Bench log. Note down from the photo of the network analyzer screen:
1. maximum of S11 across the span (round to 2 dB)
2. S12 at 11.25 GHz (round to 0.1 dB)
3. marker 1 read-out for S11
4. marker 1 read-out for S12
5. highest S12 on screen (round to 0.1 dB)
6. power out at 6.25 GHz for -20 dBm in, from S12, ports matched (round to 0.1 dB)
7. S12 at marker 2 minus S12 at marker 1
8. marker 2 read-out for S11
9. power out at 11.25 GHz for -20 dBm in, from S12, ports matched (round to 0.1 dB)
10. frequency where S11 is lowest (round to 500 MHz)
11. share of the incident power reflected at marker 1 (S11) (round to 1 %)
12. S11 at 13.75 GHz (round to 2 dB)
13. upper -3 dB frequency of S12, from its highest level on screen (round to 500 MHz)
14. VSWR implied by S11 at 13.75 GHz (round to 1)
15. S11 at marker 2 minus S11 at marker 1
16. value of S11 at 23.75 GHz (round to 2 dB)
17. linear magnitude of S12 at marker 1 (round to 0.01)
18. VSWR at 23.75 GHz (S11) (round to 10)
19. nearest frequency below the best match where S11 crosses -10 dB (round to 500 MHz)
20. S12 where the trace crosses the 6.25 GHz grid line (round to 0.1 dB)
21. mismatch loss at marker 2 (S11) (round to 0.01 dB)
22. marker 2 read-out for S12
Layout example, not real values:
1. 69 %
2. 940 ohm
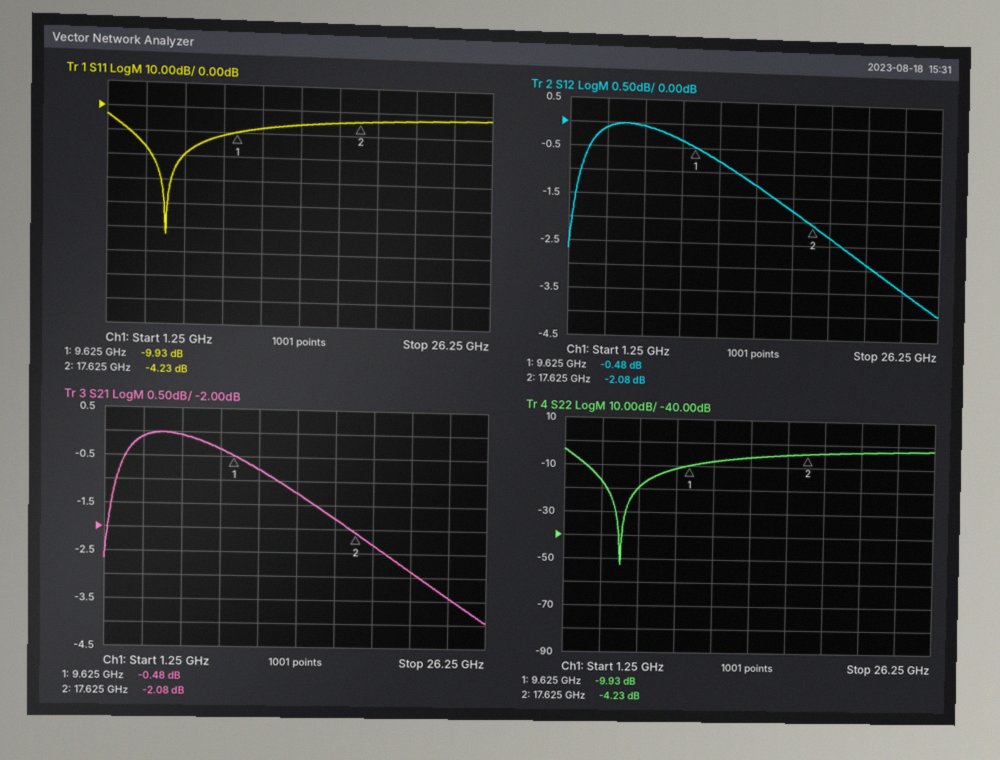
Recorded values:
1. -2 dB
2. -0.8 dB
3. -9.93 dB
4. -0.48 dB
5. 0.0 dB
6. -20.1 dBm
7. -1.60 dB
8. -4.23 dB
9. -20.8 dBm
10. 5.0 GHz
11. 10 %
12. -6 dB
13. 22.0 GHz
14. 3
15. 5.70 dB
16. -2 dB
17. 0.95
18. 10
19. 2.5 GHz
20. -0.1 dB
21. 2.06 dB
22. -2.08 dB
